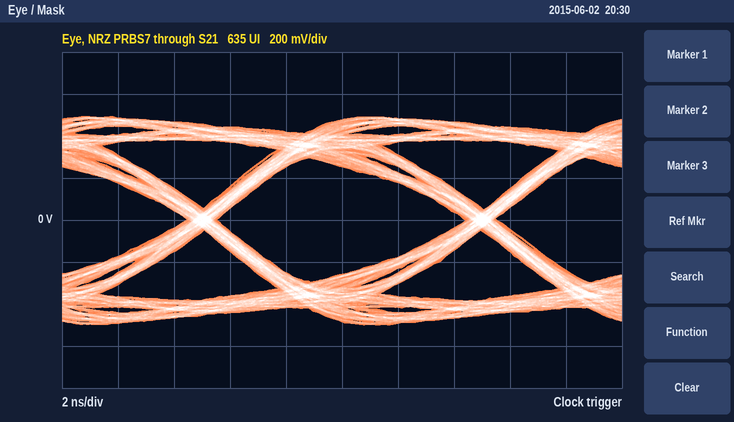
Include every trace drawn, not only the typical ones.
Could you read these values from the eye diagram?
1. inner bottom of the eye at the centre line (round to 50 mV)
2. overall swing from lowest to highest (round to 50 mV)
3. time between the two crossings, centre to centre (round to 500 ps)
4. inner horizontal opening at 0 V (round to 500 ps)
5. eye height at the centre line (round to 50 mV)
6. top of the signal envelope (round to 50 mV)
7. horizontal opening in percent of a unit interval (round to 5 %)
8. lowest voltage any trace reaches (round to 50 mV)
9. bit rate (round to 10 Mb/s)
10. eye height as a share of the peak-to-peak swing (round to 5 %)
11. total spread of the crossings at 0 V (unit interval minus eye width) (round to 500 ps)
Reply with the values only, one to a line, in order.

-250 mV
1.00 V
10.0 ns
9.0 ns
500 mV
500 mV
90 %
-500 mV
100 Mb/s
50 %
1.0 ns
